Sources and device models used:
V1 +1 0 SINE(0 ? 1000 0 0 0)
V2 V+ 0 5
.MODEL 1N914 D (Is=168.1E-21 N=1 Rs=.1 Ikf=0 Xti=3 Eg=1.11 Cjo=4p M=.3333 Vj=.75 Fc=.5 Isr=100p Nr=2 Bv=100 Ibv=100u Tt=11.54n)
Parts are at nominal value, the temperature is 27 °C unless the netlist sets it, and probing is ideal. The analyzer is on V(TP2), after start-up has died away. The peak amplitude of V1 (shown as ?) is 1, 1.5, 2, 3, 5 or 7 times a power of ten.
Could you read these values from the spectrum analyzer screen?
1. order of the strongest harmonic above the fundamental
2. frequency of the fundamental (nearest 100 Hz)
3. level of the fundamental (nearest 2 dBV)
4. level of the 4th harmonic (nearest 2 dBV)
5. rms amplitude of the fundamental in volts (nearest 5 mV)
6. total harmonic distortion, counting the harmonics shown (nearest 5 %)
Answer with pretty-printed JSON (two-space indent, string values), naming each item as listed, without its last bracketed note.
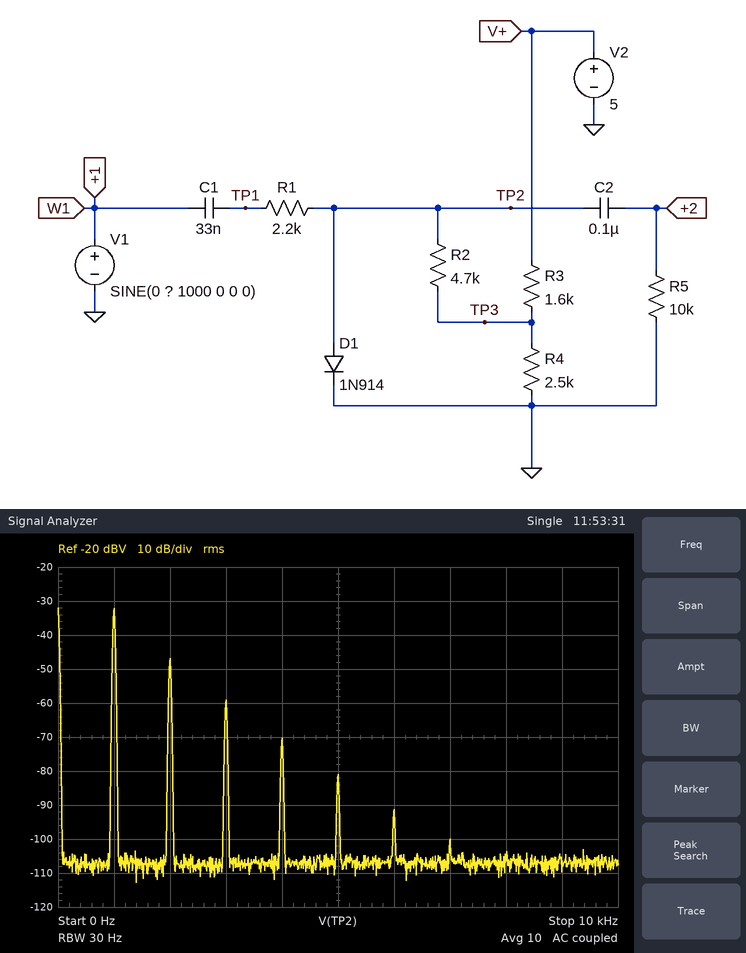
{
  "order of the strongest harmonic above the fundamental": "2",
  "frequency of the fundamental": "1.0 kHz",
  "level of the fundamental": "-32 dBV",
  "level of the 4th harmonic": "-70 dBV",
  "rms amplitude of the fundamental in volts": "25 mV",
  "total harmonic distortion, counting the harmonics shown": "20 %"
}
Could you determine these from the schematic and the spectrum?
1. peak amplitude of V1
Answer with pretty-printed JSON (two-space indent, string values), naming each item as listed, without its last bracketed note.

{
  "peak amplitude of V1": "1.5 V"
}
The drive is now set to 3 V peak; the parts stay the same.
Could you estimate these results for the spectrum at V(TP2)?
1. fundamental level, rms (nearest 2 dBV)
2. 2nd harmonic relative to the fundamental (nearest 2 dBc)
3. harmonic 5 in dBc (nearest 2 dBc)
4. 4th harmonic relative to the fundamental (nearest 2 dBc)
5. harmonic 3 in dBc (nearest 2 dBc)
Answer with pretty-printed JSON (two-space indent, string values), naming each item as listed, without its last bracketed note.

{
  "fundamental level, rms": "-18 dBV",
  "2nd harmonic relative to the fundamental": "-6 dBc",
  "harmonic 5 in dBc": "-32 dBc",
  "4th harmonic relative to the fundamental": "-20 dBc",
  "harmonic 3 in dBc": "-12 dBc"
}
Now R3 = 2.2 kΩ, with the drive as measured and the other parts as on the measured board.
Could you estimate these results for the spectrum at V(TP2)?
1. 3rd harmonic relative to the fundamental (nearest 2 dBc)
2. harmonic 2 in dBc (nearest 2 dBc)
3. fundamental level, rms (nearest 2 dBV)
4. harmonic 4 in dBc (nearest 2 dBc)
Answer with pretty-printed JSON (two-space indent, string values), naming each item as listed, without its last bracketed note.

{
  "3rd harmonic relative to the fundamental": "-22 dBc",
  "harmonic 2 in dBc": "-12 dBc",
  "fundamental level, rms": "-30 dBV",
  "harmonic 4 in dBc": "-30 dBc"
}
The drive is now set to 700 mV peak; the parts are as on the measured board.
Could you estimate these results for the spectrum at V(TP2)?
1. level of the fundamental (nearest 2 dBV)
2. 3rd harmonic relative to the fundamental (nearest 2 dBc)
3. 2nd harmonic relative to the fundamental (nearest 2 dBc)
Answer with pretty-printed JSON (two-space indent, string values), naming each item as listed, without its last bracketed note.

{
  "level of the fundamental": "-40 dBV",
  "3rd harmonic relative to the fundamental": "-42 dBc",
  "2nd harmonic relative to the fundamental": "-22 dBc"
}
